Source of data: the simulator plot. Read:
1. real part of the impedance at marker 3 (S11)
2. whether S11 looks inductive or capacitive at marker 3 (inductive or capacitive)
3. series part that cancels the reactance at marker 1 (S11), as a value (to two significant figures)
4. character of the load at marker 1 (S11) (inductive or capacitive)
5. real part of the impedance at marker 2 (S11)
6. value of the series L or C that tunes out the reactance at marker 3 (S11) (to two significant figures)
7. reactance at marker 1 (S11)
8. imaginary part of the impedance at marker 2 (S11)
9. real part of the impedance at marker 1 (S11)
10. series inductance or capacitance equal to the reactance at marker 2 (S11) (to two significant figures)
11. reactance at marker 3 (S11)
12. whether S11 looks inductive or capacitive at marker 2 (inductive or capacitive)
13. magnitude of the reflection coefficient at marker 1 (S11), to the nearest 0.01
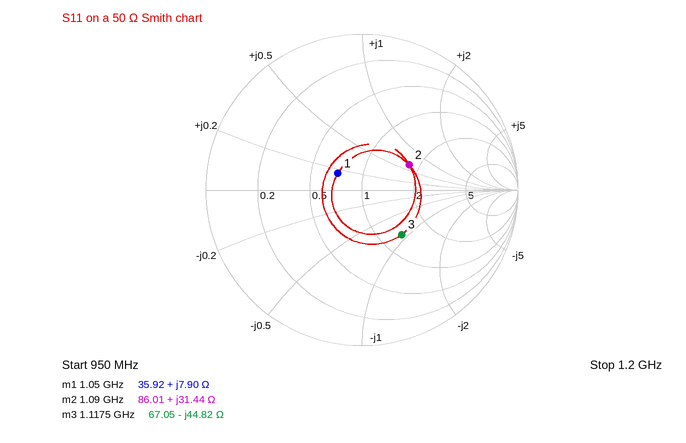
67.05 Ω
capacitive
19 pF
inductive
86.01 Ω
6.4 nH
+7.90 Ω
+31.44 Ω
35.92 Ω
4.6 nH
-44.82 Ω
inductive
0.19
